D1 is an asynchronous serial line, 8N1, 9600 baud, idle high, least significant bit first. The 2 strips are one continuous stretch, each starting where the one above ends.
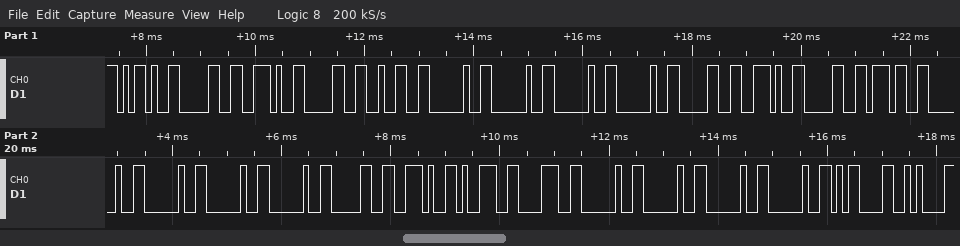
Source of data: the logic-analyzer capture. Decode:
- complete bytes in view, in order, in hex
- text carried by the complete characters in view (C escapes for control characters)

2D 30 2E 30 32 20 20 20 20 30 2E 30 37 20 20 20 20 30 2E 39 38 20 20 20 20 0D 0A
"-0.02    0.07    0.98    \r\n"
